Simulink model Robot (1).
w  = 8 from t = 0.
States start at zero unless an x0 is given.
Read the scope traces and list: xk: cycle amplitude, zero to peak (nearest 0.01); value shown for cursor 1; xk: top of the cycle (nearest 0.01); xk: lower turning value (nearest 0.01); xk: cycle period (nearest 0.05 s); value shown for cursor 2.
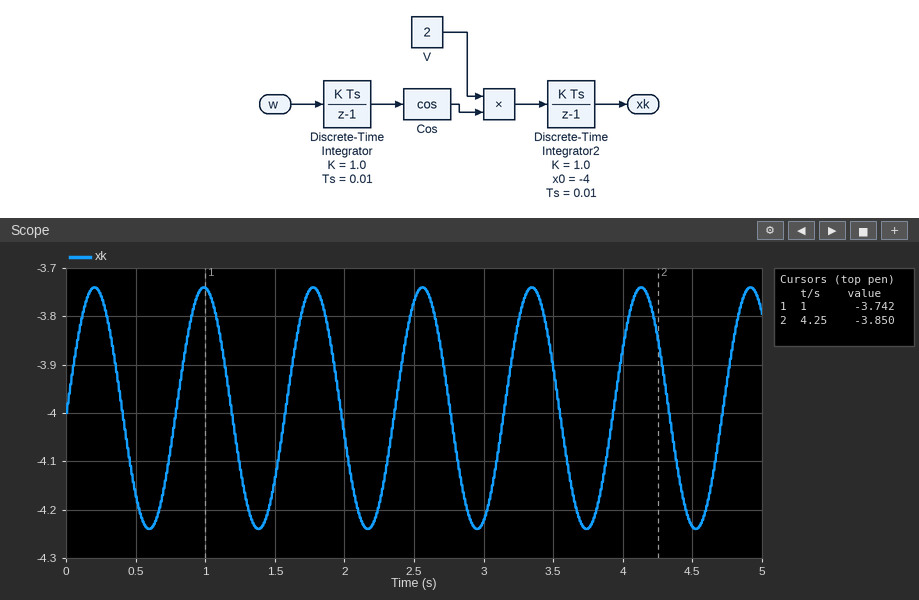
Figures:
0.25
-3.742
-3.74
-4.24
0.80 s
-3.850
